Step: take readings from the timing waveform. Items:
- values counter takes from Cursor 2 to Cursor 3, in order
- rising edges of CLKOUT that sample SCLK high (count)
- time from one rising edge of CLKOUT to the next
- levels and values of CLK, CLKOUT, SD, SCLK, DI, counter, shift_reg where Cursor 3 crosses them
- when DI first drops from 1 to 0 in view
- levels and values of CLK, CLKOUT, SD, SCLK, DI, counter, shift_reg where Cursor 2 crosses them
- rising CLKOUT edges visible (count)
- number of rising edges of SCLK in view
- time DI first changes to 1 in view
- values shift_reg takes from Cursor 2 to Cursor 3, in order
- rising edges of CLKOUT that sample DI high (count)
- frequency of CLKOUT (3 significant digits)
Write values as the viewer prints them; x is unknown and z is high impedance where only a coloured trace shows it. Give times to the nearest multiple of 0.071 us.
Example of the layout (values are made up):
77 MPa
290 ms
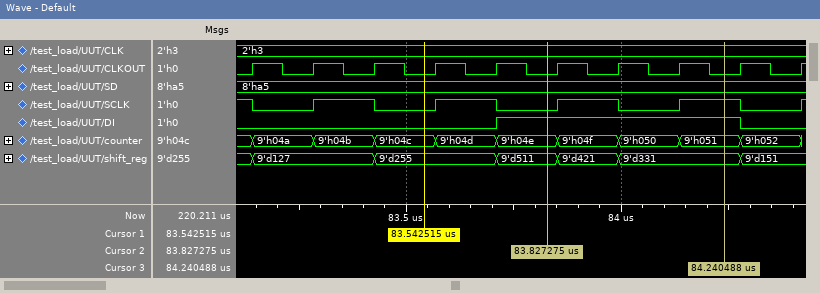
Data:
9'h04e, 9'h04f, 9'h050, 9'h051
5
0.142 us
CLK=2'h3, CLKOUT=0, SD=8'ha5, SCLK=1, DI=1, counter=9'h051, shift_reg=9'd331
84.277 us
CLK=2'h3, CLKOUT=0, SD=8'ha5, SCLK=0, DI=1, counter=9'h04e, shift_reg=9'd511
10
5
83.709 us
9'd511, 9'd421, 9'd331
4
7.04 MHz
